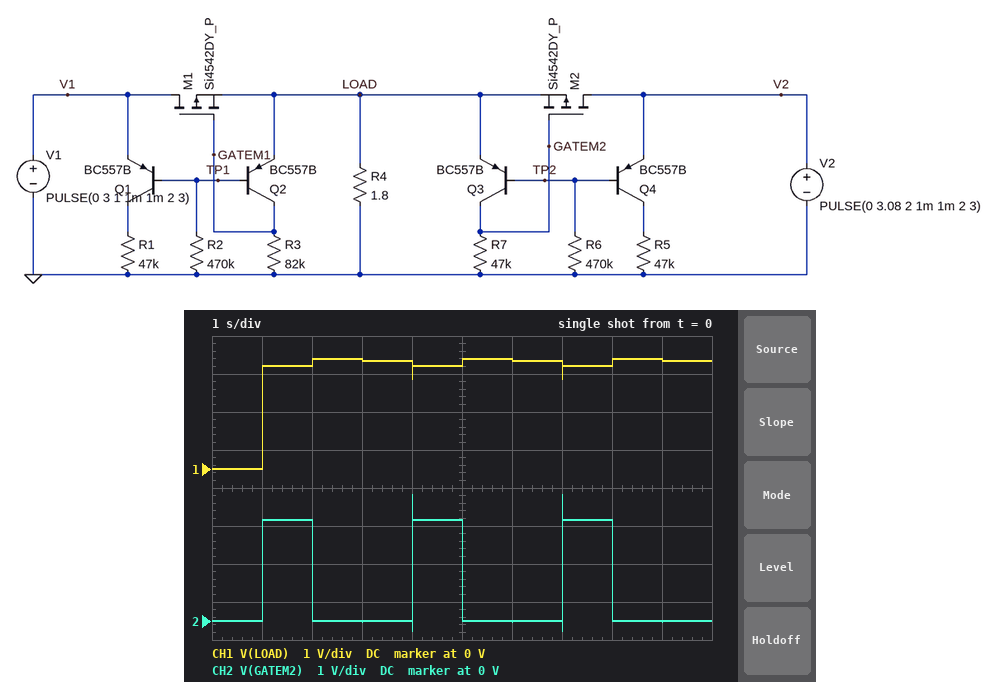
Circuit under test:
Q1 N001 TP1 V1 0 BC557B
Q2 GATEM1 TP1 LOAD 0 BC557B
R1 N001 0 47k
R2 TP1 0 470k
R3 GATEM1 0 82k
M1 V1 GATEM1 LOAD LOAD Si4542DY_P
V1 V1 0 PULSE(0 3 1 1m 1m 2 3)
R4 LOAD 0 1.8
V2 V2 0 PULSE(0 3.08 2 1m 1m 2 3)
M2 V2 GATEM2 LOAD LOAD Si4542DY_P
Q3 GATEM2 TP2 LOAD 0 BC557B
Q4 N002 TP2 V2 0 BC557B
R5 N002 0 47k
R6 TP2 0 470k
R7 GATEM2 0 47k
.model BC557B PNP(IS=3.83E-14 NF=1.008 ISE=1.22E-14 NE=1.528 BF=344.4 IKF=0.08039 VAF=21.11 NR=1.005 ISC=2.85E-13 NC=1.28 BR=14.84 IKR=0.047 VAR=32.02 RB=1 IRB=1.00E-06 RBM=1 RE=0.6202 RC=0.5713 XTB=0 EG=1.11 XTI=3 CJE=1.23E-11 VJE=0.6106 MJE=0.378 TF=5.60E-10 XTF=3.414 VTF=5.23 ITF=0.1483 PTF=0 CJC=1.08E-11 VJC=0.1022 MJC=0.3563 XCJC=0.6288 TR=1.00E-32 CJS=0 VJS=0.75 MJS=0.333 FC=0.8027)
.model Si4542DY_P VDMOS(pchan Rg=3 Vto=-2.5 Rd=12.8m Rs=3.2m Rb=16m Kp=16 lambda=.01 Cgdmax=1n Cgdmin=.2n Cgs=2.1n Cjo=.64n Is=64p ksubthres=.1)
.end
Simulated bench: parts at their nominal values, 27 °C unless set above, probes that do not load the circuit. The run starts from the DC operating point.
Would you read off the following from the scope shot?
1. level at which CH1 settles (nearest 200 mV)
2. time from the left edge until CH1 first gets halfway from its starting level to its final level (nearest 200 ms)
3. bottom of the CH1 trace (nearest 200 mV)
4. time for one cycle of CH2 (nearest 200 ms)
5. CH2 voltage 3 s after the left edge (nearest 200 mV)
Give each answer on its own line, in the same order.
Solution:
2.8 V
1.0 s
0 V
3.0 s
0 V
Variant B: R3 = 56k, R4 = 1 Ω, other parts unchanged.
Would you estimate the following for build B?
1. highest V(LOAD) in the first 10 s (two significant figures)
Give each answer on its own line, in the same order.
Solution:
2.8 V
